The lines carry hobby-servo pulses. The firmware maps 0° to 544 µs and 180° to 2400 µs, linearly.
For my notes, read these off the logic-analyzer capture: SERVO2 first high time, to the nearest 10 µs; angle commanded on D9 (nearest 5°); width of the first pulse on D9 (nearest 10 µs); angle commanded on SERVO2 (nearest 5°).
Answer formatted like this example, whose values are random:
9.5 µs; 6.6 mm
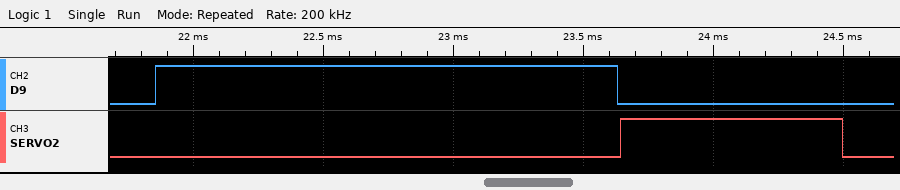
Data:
850 µs; 120°; 1780 µs; 30°
